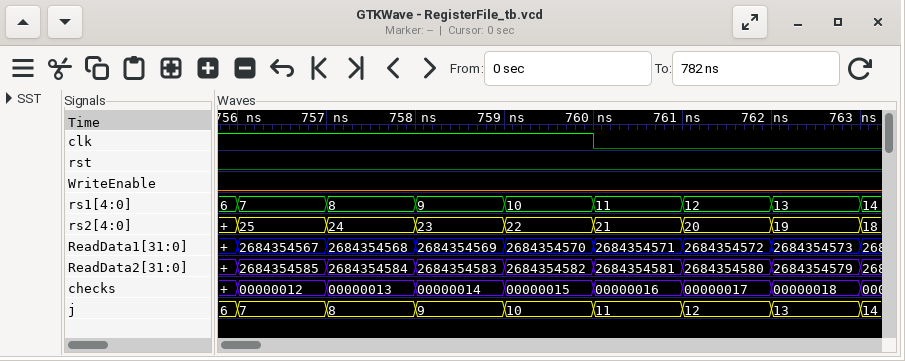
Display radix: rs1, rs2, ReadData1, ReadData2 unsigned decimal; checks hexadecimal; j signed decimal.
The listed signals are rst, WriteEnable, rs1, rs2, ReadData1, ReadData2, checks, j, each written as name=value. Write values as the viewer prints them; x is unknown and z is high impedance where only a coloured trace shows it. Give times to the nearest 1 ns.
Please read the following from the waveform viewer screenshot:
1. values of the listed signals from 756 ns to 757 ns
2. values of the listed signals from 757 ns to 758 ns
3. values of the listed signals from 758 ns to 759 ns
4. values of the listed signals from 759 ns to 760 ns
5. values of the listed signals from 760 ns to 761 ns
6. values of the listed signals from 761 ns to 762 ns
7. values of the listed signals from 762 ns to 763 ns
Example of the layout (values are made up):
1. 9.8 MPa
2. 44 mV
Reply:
1. rst=0, WriteEnable=0, rs1=7, rs2=25, ReadData1=2684354567, ReadData2=2684354585, checks=00000012, j=7
2. rst=0, WriteEnable=0, rs1=8, rs2=24, ReadData1=2684354568, ReadData2=2684354584, checks=00000013, j=8
3. rst=0, WriteEnable=0, rs1=9, rs2=23, ReadData1=2684354569, ReadData2=2684354583, checks=00000014, j=9
4. rst=0, WriteEnable=0, rs1=10, rs2=22, ReadData1=2684354570, ReadData2=2684354582, checks=00000015, j=10
5. rst=0, WriteEnable=0, rs1=11, rs2=21, ReadData1=2684354571, ReadData2=2684354581, checks=00000016, j=11
6. rst=0, WriteEnable=0, rs1=12, rs2=20, ReadData1=2684354572, ReadData2=2684354580, checks=00000017, j=12
7. rst=0, WriteEnable=0, rs1=13, rs2=19, ReadData1=2684354573, ReadData2=2684354579, checks=00000018, j=13
